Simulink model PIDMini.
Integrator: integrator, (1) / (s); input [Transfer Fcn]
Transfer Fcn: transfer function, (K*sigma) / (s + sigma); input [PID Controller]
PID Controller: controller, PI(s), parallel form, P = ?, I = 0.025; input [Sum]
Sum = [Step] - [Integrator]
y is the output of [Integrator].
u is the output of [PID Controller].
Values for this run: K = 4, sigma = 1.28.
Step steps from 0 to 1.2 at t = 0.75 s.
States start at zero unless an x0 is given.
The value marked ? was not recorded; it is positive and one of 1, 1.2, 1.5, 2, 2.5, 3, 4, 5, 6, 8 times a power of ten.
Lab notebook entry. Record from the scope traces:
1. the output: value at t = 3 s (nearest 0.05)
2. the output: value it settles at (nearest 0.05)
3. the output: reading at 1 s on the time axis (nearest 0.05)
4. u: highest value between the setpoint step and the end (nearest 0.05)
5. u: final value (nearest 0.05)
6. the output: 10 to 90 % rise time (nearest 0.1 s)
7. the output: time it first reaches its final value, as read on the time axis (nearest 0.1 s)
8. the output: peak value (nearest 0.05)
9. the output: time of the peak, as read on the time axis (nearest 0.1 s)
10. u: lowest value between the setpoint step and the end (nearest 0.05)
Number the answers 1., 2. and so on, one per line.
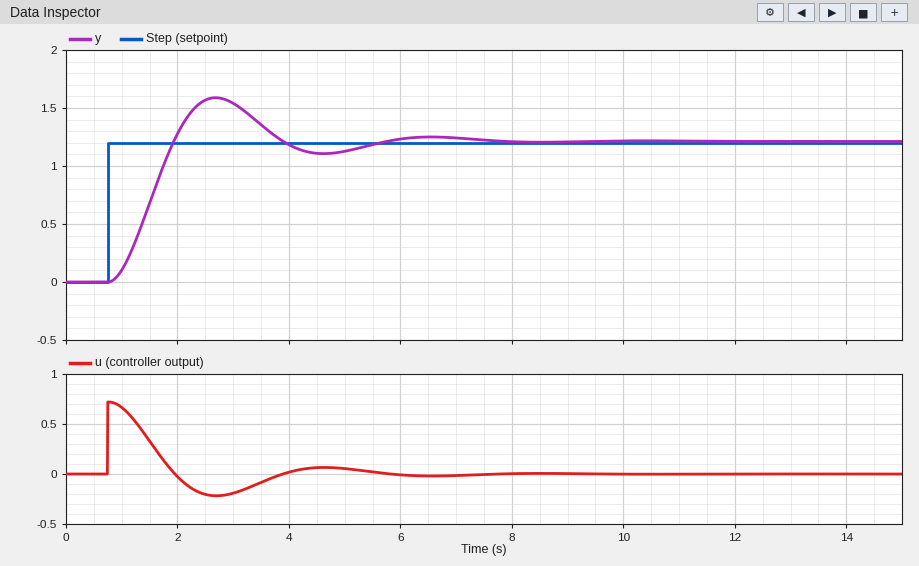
1. 1.55
2. 1.20
3. 0.10
4. 0.70
5. 0.00
6. 0.8 s
7. 1.9 s
8. 1.60
9. 2.7 s
10. -0.20
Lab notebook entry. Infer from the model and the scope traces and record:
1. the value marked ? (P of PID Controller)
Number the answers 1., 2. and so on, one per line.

1. 0.6
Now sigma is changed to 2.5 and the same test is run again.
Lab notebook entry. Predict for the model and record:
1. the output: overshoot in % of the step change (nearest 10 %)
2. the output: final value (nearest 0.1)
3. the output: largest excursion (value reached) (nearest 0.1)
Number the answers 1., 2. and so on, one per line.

1. 20 %
2. 1.2
3. 1.4
